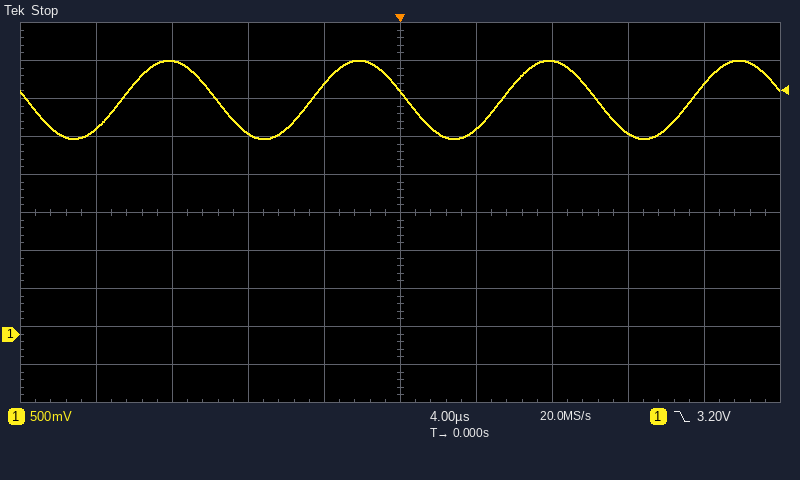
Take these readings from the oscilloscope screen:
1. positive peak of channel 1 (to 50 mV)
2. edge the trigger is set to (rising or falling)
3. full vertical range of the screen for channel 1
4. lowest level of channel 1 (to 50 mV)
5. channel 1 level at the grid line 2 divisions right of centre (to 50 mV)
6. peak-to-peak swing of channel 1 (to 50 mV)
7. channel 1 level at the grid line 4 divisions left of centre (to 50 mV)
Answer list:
3.60 V
falling
5 V
2.55 V
3.60 V
1.05 V
2.70 V
